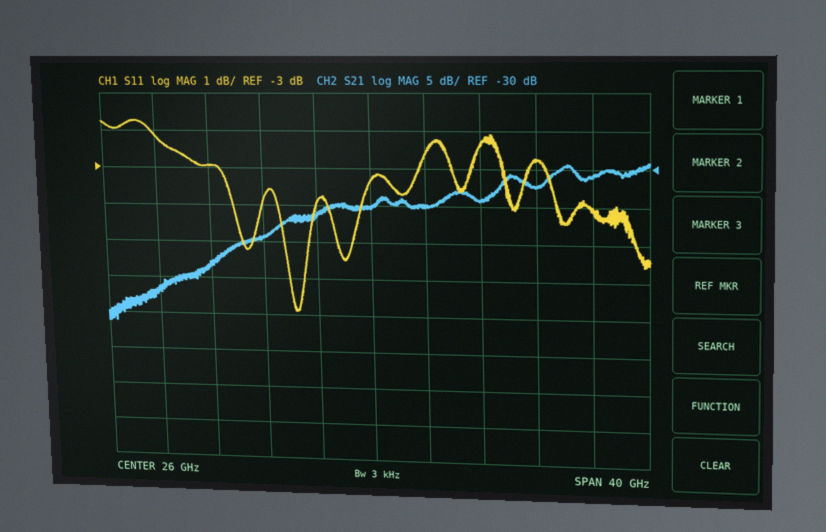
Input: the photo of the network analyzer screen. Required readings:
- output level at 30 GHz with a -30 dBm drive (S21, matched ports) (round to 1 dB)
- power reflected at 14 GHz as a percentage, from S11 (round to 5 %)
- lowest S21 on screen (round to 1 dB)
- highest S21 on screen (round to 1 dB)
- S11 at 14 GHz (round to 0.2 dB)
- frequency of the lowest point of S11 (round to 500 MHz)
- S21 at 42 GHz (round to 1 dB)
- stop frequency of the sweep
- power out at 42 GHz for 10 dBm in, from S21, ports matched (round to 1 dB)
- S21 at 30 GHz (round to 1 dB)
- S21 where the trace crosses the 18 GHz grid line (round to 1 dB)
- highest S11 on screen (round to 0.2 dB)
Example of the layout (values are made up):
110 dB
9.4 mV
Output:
-65 dBm
50 %
-51 dB
-29 dB
-3.0 dB
20.5 GHz
-31 dB
46 GHz
-21 dBm
-35 dB
-39 dB
-1.8 dB
